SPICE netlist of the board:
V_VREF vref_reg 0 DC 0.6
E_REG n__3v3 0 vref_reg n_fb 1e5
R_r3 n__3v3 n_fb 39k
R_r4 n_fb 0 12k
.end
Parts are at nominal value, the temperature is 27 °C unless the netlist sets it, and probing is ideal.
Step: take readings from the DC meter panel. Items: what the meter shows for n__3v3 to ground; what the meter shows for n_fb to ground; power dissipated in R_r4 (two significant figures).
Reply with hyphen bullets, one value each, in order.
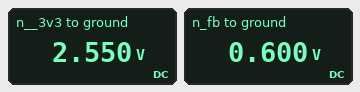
- 2.550 V
- 0.600 V
- 30 µW
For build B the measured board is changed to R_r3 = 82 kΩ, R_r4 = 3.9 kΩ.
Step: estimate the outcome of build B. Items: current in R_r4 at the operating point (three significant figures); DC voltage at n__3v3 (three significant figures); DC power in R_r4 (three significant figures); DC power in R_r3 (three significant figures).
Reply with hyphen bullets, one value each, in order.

- 154 µA
- 13.2 V
- 92.3 µW
- 1.94 mW
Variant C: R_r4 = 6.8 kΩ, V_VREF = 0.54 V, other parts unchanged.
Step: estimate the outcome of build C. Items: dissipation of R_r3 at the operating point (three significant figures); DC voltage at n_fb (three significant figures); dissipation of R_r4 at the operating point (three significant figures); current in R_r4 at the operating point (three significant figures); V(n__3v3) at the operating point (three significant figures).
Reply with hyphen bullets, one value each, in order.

- 246 µW
- 540 mV
- 42.9 µW
- 79.4 µA
- 3.64 V
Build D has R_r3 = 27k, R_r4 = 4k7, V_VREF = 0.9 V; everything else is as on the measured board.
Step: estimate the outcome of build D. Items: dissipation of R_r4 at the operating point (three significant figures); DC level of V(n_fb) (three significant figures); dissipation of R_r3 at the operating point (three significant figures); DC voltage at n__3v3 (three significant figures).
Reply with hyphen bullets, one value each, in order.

- 172 µW
- 900 mV
- 990 µW
- 6.07 V
